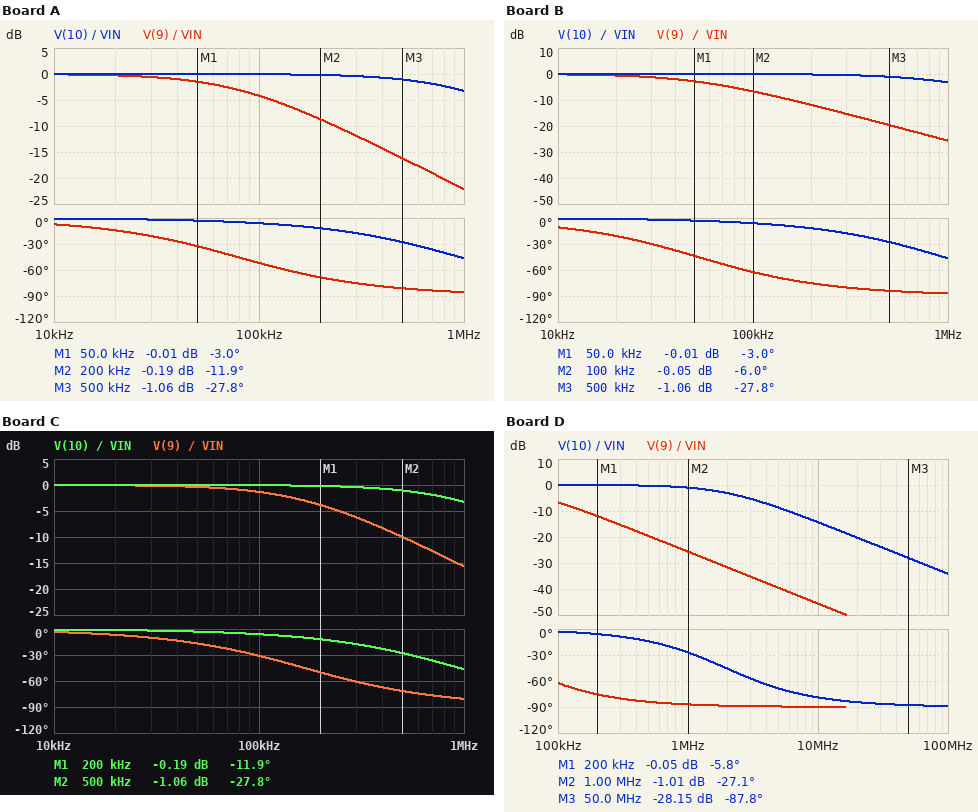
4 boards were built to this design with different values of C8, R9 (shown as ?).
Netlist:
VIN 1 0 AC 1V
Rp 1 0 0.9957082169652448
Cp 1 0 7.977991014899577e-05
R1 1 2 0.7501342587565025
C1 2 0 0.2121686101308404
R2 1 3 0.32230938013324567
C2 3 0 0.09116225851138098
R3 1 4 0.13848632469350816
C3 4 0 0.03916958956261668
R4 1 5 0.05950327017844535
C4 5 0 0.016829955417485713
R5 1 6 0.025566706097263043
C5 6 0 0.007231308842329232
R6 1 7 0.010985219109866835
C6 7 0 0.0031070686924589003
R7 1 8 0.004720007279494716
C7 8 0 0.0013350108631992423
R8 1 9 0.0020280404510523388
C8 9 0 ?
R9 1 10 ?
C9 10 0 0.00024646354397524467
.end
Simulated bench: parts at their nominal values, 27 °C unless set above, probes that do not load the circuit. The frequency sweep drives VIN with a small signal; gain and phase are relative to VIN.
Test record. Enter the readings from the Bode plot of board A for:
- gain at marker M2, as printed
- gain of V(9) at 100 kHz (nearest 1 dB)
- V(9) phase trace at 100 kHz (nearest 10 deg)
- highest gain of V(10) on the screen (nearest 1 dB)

-0.19 dB
-4 dB
-50 deg
0 dB
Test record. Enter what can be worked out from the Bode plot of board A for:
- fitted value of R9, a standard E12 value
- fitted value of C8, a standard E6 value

680 µΩ
1 mF
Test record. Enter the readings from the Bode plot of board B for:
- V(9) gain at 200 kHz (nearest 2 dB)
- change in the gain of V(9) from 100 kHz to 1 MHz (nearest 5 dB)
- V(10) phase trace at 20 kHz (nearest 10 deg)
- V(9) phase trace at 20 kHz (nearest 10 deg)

-12 dB
-20 dB
0 deg
-20 deg
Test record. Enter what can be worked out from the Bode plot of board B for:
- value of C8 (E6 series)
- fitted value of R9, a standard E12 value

1.5 mF
680 µΩ
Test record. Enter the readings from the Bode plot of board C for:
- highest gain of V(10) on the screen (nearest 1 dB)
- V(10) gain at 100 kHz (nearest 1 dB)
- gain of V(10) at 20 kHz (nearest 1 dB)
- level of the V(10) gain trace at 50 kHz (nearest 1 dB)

0 dB
0 dB
0 dB
0 dB
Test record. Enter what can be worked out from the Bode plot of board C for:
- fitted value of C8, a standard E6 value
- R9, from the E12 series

470 µF
680 µΩ
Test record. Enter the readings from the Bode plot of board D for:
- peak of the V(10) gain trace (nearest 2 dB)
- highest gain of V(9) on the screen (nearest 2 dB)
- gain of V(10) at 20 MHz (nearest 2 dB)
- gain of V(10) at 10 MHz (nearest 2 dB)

0 dB
-6 dB
-20 dB
-14 dB
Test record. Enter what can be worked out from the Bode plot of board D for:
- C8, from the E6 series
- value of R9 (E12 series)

1.5 mF
330 µΩ
